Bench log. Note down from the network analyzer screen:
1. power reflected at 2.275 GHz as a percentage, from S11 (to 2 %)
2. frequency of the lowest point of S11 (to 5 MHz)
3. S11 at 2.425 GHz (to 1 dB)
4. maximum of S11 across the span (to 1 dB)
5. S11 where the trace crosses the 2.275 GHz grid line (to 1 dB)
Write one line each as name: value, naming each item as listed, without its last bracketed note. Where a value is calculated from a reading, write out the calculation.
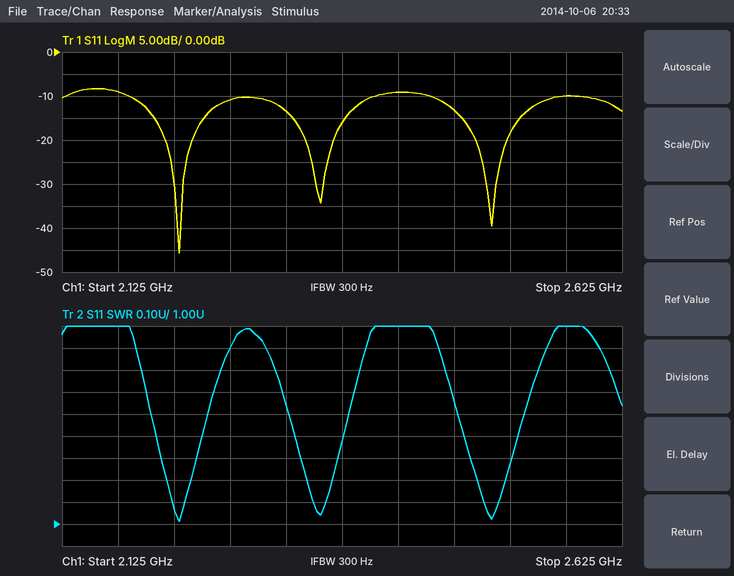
power reflected at 2.275 GHz as a percentage, from S11: 10^(-11/10) ≈ 8 %
frequency of the lowest point of S11: 2.230 GHz
S11 at 2.425 GHz: -9 dB
maximum of S11 across the span: -8 dB
S11 where the trace crosses the 2.275 GHz grid line: -11 dB
